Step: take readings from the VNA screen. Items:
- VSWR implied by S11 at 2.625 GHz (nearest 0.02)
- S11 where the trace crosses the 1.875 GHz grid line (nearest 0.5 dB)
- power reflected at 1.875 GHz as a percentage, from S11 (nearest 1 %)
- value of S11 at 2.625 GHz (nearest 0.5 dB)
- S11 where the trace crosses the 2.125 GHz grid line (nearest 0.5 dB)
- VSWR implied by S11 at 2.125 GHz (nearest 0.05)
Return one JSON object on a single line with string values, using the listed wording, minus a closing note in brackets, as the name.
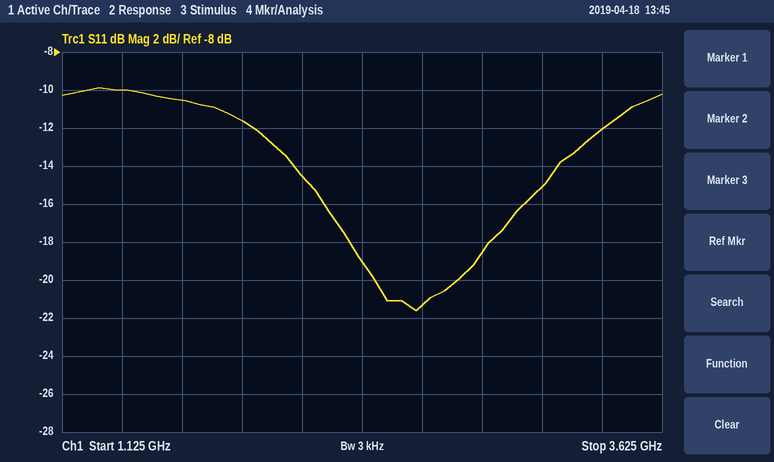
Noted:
{"VSWR implied by S11 at 2.625 GHz": "1.18", "S11 where the trace crosses the 1.875 GHz grid line": "-11.5 dB", "power reflected at 1.875 GHz as a percentage, from S11": "7 %", "value of S11 at 2.625 GHz": "-21.5 dB", "S11 where the trace crosses the 2.125 GHz grid line": "-14.5 dB", "VSWR implied by S11 at 2.125 GHz": "1.45"}
